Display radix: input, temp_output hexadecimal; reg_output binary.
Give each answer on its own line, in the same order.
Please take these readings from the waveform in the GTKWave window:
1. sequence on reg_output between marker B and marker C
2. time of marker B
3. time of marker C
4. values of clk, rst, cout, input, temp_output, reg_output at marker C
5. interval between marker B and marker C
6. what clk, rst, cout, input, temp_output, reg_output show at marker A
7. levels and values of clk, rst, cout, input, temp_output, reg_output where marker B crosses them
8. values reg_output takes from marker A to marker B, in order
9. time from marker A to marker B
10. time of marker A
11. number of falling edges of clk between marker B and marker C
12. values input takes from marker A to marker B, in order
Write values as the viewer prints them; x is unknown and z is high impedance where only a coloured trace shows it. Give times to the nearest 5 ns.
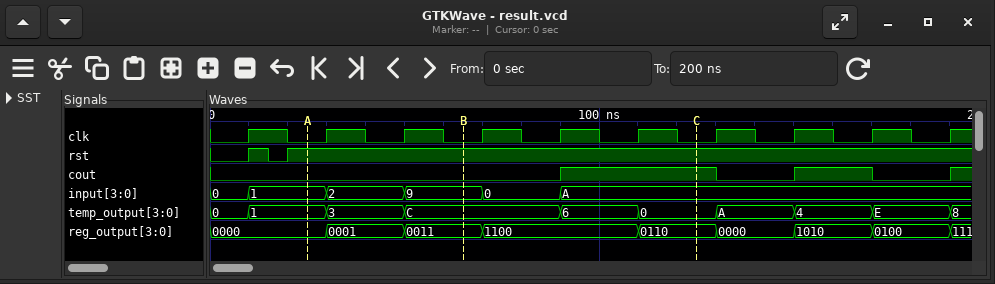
0011, 1100, 0110
65 ns
125 ns
clk=0, rst=1, cout=1, input=A, temp_output=0, reg_output=0110
60 ns
clk=0, rst=1, cout=0, input=1, temp_output=1, reg_output=0000
clk=0, rst=1, cout=0, input=9, temp_output=C, reg_output=0011
0000, 0001, 0011
40 ns
25 ns
3
1, 2, 9
